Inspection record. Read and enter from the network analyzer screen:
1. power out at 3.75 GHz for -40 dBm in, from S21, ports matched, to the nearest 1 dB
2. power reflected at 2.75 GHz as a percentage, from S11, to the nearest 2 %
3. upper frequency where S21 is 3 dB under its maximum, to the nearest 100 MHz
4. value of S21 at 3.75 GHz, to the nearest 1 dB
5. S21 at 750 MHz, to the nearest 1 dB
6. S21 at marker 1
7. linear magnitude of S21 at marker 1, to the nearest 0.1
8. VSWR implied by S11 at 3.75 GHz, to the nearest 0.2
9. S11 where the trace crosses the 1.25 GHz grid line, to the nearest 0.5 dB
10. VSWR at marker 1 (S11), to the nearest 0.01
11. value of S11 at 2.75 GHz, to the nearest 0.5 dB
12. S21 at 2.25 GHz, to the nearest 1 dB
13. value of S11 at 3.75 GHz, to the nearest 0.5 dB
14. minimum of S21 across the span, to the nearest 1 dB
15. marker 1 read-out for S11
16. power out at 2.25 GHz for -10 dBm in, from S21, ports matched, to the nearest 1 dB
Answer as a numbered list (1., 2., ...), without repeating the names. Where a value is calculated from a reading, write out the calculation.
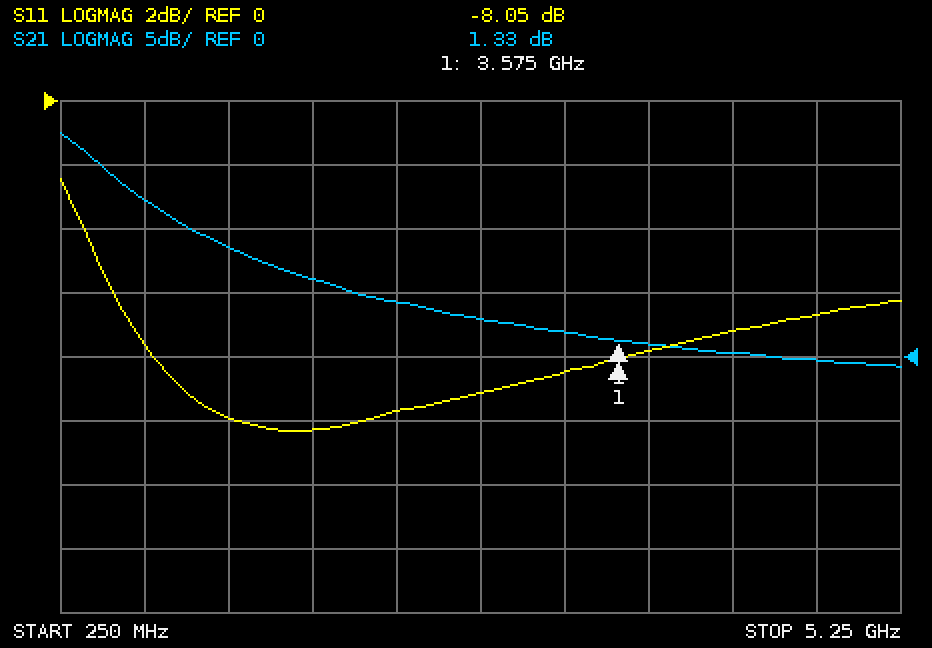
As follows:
1. -40 dBm + (1 dB) = -39 dBm
2. 10^(-9/10) ≈ 12.6 %, so 12 % to the nearest 2 %
3. 500 MHz
4. 1 dB
5. 12 dB
6. 1.33 dB
7. 10^(1.33/20) ≈ 1.2
8. |Γ| = 10^(-8/20) = 0.3981; VSWR = (1 + 0.3981)/(1 − 0.3981) ≈ 2.32, so 2.4 to the nearest 0.2
9. -10.0 dB
10. (1 + 0.3958)/(1 − 0.3958) ≈ 2.31
11. -9.0 dB
12. 4 dB
13. -8.0 dB
14. -1 dB
15. -8.05 dB
16. -10 dBm + (4 dB) = -6 dBm
